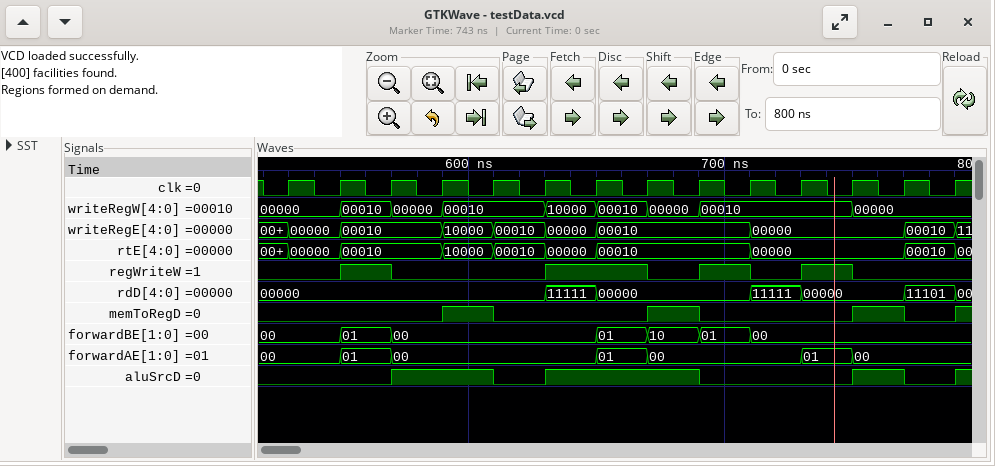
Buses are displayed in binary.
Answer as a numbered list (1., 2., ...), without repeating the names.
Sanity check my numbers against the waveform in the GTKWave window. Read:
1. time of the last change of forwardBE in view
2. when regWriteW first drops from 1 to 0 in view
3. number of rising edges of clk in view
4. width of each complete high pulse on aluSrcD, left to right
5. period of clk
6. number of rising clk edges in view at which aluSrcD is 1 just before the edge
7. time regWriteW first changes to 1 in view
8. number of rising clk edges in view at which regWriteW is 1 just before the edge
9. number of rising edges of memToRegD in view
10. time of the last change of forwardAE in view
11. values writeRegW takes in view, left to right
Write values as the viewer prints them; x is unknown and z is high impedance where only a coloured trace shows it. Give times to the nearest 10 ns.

1. 710 ns
2. 570 ns
3. 14
4. 40 ns, 60 ns, 20 ns
5. 20 ns
6. 6
7. 550 ns
8. 5
9. 4
10. 750 ns
11. 00000, 00010, 00000, 00010, 10000, 00010, 00000, 00010, 00000
